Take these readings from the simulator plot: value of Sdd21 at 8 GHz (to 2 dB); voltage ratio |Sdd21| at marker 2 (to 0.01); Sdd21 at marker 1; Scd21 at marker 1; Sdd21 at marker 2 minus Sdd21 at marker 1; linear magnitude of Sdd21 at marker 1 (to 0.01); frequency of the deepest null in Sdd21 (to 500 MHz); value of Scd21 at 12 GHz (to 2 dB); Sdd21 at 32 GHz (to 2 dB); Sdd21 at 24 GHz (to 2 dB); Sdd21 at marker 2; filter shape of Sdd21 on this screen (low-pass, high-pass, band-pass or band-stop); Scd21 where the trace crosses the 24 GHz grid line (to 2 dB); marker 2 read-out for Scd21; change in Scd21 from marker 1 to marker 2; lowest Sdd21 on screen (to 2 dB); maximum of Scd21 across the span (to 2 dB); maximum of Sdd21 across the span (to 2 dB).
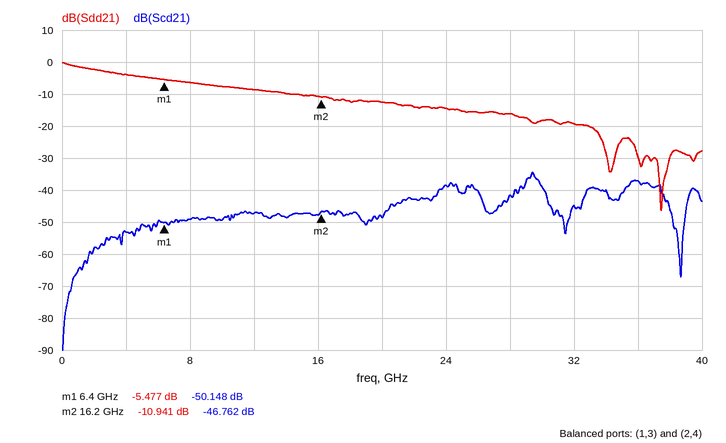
-6 dB
0.28
-5.477 dB
-50.148 dB
-5.464 dB
0.53
37.5 GHz
-48 dB
-20 dB
-14 dB
-10.941 dB
low-pass
-38 dB
-46.762 dB
3.386 dB
-46 dB
-34 dB
0 dB
